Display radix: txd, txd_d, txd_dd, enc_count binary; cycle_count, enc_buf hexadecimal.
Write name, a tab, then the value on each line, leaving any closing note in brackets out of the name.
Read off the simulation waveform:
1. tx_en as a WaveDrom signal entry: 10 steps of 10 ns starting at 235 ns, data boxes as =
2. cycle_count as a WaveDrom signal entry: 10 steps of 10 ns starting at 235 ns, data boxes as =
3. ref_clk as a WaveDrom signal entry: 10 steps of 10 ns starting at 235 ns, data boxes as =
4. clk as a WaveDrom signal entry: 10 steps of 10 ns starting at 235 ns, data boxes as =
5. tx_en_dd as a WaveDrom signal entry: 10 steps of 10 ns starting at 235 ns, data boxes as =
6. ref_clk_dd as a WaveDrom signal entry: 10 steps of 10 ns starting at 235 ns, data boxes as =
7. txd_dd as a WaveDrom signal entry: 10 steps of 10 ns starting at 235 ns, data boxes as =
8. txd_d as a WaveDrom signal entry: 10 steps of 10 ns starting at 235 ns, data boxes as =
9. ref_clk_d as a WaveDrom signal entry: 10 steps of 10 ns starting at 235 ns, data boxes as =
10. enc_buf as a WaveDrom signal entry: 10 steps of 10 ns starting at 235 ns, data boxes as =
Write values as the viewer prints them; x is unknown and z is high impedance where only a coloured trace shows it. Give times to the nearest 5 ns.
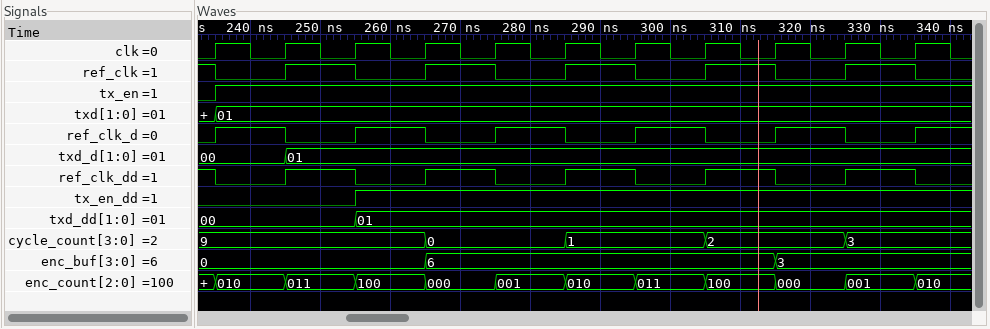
tx_en as a WaveDrom signal entry: 10 steps of 10 ns starting at 235 ns, data boxes as =	{name: 'tx_en', wave: '1.........'}
cycle_count as a WaveDrom signal entry: 10 steps of 10 ns starting at 235 ns, data boxes as =	{name: 'cycle_count', wave: '=..=.=.=.=', data: '9 0 1 2 3'}
ref_clk as a WaveDrom signal entry: 10 steps of 10 ns starting at 235 ns, data boxes as =	{name: 'ref_clk', wave: '0101010101'}
clk as a WaveDrom signal entry: 10 steps of 10 ns starting at 235 ns, data boxes as =	{name: 'clk', wave: 'p.........'}
tx_en_dd as a WaveDrom signal entry: 10 steps of 10 ns starting at 235 ns, data boxes as =	{name: 'tx_en_dd', wave: '0.1.......'}
ref_clk_dd as a WaveDrom signal entry: 10 steps of 10 ns starting at 235 ns, data boxes as =	{name: 'ref_clk_dd', wave: '0101010101'}
txd_dd as a WaveDrom signal entry: 10 steps of 10 ns starting at 235 ns, data boxes as =	{name: 'txd_dd', wave: '=.=.......', data: '00 01'}
txd_d as a WaveDrom signal entry: 10 steps of 10 ns starting at 235 ns, data boxes as =	{name: 'txd_d', wave: '==........', data: '00 01'}
ref_clk_d as a WaveDrom signal entry: 10 steps of 10 ns starting at 235 ns, data boxes as =	{name: 'ref_clk_d', wave: '1010101010'}
enc_buf as a WaveDrom signal entry: 10 steps of 10 ns starting at 235 ns, data boxes as =	{name: 'enc_buf', wave: '=..=....=.', data: '0 6 3'}
